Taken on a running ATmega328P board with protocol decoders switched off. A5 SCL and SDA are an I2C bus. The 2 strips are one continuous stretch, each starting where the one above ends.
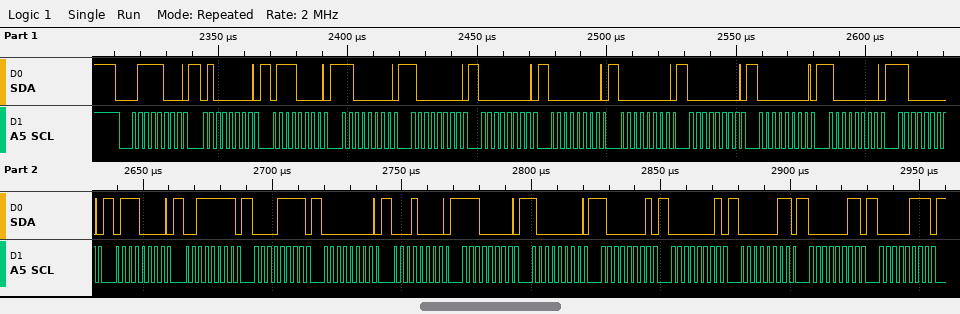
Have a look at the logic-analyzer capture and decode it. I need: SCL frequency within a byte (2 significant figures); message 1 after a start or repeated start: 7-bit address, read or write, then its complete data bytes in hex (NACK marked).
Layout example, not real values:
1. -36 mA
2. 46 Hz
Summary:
1. 400 kHz
2. 0x3C write: 40 70 C0 80 00 00 00 00 00 80 C0 70 3F 0F 00 10 E0 80 81 01 03 03 07
